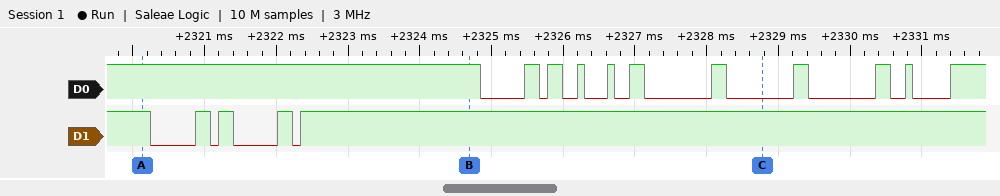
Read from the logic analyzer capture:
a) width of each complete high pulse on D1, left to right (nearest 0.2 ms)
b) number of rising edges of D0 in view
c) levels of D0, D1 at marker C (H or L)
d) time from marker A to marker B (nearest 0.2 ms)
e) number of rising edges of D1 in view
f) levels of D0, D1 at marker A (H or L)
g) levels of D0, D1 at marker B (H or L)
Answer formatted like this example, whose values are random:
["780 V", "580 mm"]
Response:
["0.2 ms, 0.2 ms, 0.2 ms", "10", "D0=L, D1=H", "4.6 ms", "4", "D0=H, D1=H", "D0=H, D1=H"]
